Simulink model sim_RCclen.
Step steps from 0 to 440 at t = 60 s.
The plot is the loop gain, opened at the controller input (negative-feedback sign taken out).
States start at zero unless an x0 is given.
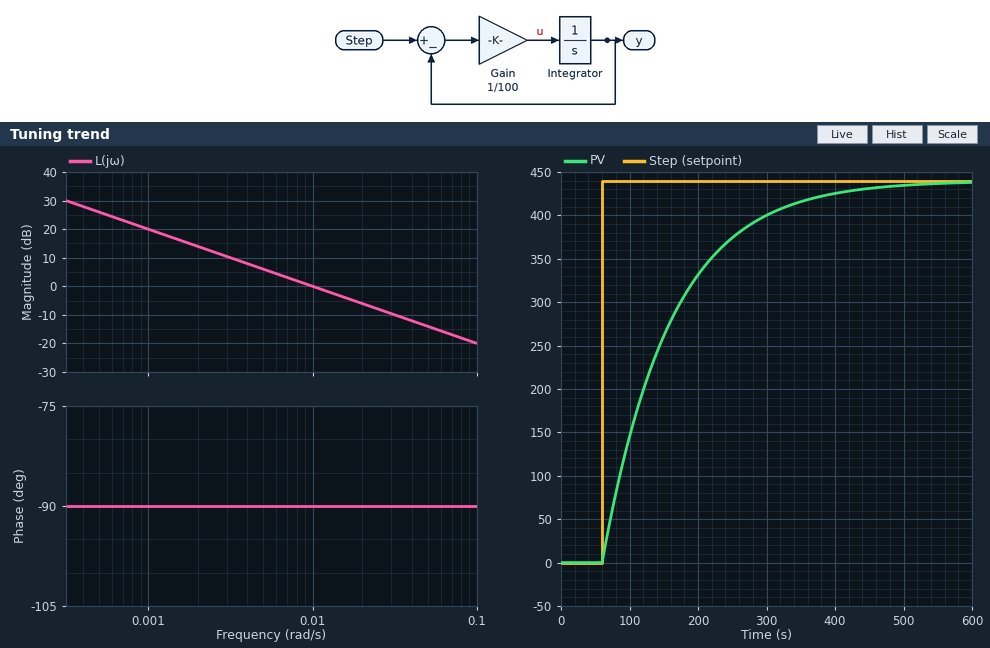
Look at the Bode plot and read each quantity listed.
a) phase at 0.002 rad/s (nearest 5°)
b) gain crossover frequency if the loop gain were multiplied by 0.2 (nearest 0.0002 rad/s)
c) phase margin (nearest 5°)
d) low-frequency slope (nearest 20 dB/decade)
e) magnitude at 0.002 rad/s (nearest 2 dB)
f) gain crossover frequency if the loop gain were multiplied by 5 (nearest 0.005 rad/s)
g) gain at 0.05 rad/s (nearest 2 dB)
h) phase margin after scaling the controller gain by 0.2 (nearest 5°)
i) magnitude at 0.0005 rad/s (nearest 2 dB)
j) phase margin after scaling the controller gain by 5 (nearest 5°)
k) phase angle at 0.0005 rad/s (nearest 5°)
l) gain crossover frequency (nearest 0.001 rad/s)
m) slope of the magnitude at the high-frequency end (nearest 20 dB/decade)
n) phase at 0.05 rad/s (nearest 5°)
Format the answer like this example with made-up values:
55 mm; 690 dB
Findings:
-90°; 0.0020 rad/s; 90°; -20 dB/decade; 14 dB; 0.050 rad/s; -14 dB; 90°; 26 dB; 90°; -90°; 0.010 rad/s; -20 dB/decade; -90°
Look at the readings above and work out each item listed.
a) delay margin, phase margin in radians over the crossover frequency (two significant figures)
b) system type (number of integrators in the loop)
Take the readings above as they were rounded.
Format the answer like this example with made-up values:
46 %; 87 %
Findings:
160 s; 1
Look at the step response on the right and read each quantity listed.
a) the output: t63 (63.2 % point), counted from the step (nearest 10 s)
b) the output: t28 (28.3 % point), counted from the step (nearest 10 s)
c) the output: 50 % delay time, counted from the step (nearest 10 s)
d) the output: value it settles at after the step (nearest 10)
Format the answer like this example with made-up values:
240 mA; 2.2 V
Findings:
100 s; 30 s; 70 s; 440
